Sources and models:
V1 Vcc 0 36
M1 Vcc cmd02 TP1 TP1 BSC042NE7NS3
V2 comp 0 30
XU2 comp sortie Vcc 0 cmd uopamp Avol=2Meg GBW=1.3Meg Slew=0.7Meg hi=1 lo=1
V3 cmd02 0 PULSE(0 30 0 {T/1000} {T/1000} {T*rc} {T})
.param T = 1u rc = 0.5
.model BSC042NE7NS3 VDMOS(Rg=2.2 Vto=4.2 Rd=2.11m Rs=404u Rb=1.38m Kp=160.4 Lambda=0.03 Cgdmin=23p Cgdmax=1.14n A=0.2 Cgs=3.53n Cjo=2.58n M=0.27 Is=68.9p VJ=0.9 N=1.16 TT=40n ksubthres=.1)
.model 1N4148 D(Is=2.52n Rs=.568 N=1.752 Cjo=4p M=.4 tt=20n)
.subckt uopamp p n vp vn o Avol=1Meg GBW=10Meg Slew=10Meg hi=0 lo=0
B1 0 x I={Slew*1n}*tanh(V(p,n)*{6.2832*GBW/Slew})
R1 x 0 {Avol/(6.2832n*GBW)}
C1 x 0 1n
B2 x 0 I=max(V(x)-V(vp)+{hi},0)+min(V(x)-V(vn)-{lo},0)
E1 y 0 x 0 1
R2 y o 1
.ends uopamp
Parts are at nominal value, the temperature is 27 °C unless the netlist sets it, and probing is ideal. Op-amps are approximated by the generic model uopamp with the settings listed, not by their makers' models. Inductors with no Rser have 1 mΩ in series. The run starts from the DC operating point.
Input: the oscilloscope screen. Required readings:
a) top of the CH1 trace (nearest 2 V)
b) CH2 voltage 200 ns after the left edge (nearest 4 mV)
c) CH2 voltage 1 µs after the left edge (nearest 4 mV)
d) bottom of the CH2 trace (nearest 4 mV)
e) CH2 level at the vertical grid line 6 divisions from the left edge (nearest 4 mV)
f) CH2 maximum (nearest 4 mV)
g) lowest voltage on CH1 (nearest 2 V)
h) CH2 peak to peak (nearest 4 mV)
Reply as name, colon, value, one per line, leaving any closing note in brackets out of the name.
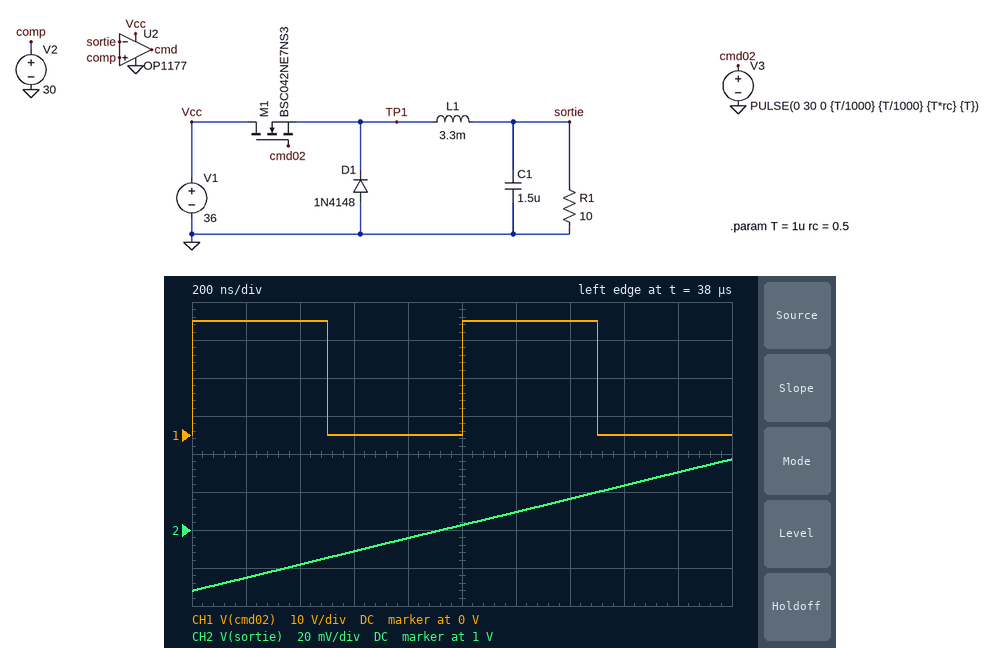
top of the CH1 trace: 30 V
CH2 voltage 200 ns after the left edge: 976 mV
CH2 voltage 1 µs after the left edge: 1.004 V
bottom of the CH2 trace: 968 mV
CH2 level at the vertical grid line 6 divisions from the left edge: 1.008 V
CH2 maximum: 1.036 V
lowest voltage on CH1: 0 V
CH2 peak to peak: 68 mV
